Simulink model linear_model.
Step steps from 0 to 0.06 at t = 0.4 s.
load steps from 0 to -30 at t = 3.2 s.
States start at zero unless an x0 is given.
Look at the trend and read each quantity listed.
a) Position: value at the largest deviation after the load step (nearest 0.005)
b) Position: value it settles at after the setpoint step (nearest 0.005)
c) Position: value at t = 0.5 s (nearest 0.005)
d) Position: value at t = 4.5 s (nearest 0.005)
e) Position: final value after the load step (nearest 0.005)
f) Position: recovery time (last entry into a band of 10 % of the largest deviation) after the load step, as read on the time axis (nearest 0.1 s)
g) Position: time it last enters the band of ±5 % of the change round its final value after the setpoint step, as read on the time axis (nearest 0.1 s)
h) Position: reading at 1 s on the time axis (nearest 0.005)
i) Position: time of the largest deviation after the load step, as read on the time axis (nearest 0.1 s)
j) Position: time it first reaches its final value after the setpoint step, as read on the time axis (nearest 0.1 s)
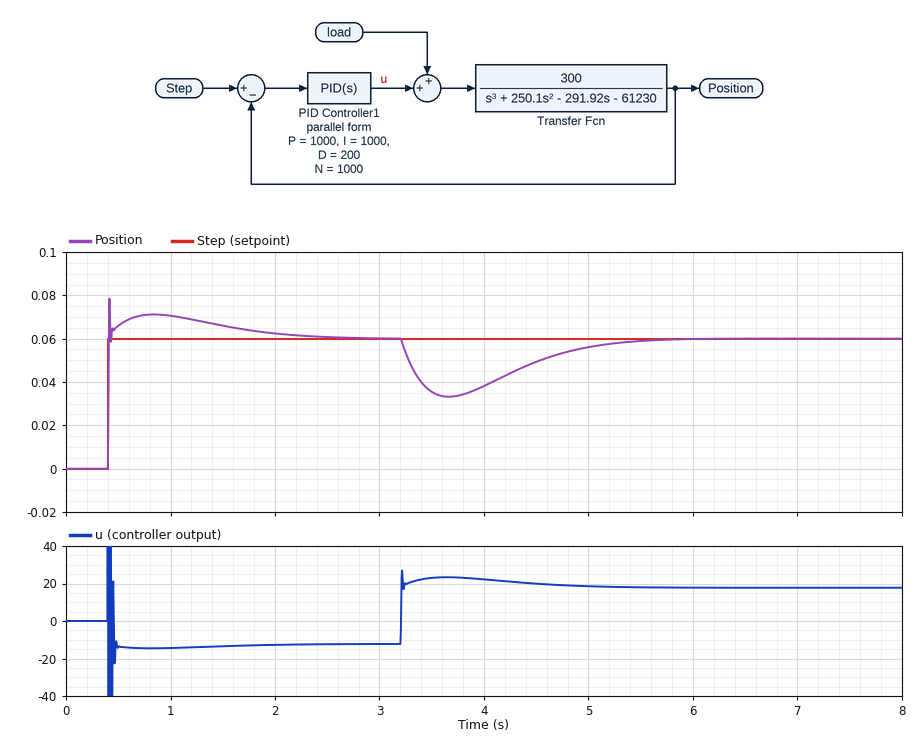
0.035
0.060
0.065
0.050
0.060
5.2 s
1.9 s
0.070
3.7 s
0.4 s
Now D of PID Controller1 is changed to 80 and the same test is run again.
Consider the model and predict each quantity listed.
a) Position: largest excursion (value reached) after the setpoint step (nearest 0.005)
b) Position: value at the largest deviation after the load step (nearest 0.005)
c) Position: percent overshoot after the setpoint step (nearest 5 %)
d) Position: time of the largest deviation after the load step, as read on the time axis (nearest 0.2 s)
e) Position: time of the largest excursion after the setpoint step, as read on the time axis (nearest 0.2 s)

0.075
0.030
25 %
3.4 s
0.6 s
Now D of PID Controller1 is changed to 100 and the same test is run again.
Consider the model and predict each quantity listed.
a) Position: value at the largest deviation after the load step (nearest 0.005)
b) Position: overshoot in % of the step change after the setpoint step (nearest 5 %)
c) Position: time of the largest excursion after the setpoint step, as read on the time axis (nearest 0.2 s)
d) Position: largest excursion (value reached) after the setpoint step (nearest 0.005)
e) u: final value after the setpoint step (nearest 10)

0.030
20 %
0.6 s
0.075
-10
